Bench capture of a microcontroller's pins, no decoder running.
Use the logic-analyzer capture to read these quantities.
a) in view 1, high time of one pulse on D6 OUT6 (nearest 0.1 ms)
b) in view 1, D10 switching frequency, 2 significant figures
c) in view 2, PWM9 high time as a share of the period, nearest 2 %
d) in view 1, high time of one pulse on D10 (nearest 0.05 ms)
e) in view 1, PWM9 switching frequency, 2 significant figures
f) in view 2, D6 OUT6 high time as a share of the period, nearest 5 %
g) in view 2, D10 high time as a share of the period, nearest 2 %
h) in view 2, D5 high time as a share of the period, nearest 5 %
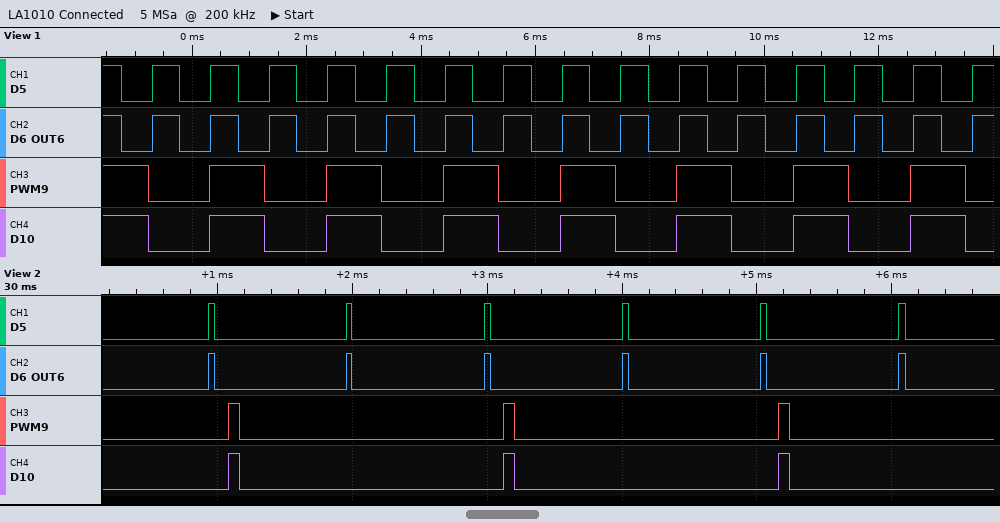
0.5 ms
490 Hz
4 %
0.95 ms
490 Hz
5 %
4 %
5 %
